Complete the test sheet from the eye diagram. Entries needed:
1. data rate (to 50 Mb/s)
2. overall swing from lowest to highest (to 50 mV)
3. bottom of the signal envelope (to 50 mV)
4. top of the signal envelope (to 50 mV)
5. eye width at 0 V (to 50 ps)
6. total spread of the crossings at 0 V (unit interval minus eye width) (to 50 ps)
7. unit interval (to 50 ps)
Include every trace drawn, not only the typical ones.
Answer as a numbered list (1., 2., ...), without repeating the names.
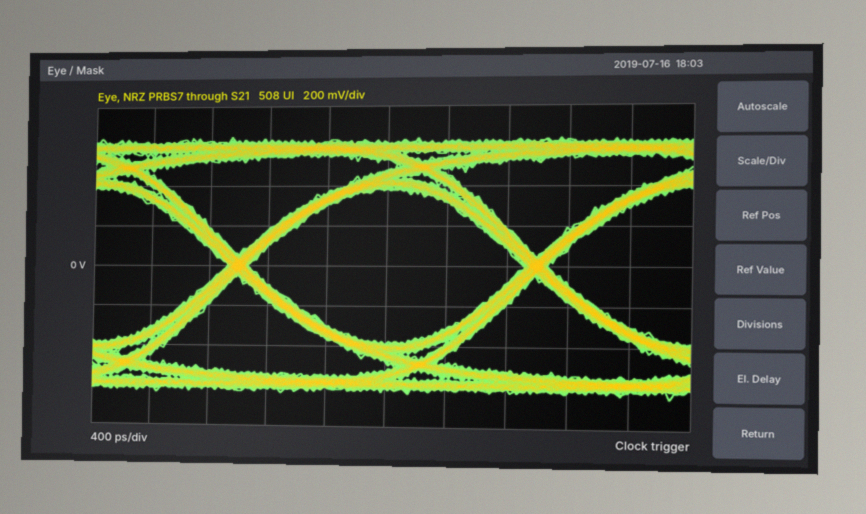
1. 500 Mb/s
2. 1.30 V
3. -650 mV
4. 650 mV
5. 1.85 ns
6. 150 ps
7. 2.00 ns
